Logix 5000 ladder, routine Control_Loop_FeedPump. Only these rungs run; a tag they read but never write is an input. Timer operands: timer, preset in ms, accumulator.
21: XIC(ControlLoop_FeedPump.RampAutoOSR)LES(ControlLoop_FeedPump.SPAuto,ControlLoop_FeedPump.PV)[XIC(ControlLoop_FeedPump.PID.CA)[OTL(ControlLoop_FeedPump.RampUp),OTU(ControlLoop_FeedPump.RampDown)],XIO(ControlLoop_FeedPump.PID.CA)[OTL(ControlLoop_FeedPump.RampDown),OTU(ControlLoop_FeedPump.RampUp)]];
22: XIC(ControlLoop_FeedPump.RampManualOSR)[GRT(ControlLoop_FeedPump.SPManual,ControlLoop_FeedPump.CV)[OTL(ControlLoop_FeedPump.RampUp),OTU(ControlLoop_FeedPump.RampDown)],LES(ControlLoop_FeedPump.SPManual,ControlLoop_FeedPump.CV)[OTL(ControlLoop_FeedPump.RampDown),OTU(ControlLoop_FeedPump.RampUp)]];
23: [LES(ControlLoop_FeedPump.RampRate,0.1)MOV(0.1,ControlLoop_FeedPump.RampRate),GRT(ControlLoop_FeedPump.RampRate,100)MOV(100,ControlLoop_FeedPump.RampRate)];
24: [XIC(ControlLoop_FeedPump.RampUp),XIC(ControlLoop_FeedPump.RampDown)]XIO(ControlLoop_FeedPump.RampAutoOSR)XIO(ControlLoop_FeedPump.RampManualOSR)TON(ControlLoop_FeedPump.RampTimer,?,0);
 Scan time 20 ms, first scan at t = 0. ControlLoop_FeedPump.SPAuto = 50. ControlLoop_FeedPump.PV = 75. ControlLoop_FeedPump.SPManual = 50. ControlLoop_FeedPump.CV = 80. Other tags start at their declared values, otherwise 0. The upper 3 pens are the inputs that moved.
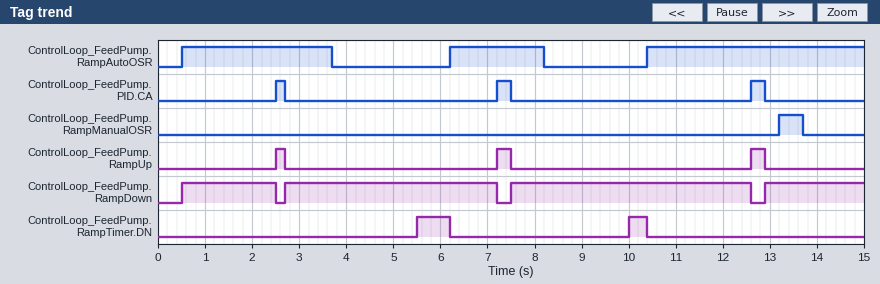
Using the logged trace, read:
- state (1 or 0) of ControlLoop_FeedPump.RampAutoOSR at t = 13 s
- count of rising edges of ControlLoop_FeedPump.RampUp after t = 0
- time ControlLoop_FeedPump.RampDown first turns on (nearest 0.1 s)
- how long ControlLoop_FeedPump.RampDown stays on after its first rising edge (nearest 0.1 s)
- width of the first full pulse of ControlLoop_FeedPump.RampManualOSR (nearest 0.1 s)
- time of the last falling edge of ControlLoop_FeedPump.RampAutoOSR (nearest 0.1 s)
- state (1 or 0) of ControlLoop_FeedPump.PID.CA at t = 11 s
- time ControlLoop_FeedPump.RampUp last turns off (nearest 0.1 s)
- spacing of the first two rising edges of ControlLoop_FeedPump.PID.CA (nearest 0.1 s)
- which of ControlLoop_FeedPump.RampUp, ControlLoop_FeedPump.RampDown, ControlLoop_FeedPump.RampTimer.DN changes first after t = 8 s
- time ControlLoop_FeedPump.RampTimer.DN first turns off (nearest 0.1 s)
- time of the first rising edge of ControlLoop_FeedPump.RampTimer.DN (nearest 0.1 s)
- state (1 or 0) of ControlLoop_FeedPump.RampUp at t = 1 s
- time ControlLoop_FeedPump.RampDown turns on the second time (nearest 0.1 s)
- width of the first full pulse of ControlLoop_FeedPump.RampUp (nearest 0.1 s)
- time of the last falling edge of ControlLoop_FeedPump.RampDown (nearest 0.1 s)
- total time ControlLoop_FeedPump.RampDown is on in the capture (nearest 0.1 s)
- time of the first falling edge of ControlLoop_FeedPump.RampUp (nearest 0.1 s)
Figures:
1
3
0.5 s
2.0 s
0.5 s
8.2 s
0
12.9 s
4.7 s
ControlLoop_FeedPump.RampTimer.DN
6.2 s
5.5 s
0
2.7 s
0.2 s
12.6 s
13.7 s
2.7 s
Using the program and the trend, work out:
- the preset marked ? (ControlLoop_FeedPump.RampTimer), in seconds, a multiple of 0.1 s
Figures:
1.8 s
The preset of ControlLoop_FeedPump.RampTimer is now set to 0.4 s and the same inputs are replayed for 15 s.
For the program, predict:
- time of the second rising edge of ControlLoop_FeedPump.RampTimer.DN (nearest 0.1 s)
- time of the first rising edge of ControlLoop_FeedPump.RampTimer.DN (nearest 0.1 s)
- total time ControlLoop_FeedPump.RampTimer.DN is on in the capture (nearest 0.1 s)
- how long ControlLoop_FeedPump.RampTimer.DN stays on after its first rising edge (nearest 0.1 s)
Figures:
8.6 s
4.1 s
3.9 s
2.1 s
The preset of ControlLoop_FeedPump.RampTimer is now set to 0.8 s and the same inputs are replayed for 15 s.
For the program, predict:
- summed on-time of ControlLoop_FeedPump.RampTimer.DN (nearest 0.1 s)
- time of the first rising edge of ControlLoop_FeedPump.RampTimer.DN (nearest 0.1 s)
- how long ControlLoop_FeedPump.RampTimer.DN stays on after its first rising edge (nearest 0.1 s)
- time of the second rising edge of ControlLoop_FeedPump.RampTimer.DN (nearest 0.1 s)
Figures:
3.1 s
4.5 s
1.7 s
9.0 s
